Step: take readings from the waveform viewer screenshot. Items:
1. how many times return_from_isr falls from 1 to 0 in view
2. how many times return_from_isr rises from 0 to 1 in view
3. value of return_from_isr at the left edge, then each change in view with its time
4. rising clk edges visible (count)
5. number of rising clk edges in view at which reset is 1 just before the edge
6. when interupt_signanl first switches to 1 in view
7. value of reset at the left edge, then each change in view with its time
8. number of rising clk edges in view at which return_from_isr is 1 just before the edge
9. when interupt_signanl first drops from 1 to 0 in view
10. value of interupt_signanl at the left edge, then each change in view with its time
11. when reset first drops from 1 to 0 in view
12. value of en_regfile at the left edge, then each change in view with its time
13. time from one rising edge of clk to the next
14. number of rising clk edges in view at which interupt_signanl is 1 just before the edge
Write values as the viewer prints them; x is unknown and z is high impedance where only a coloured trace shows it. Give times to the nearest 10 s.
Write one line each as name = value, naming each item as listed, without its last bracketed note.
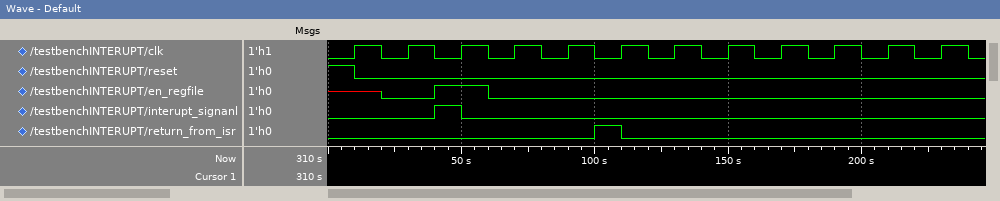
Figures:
how many times return_from_isr falls from 1 to 0 in view = 1
how many times return_from_isr rises from 0 to 1 in view = 1
value of return_from_isr at the left edge, then each change in view with its time = 0, 1 at 100 s, 0 at 110 s
rising clk edges visible = 12
number of rising clk edges in view at which reset is 1 just before the edge = 1
when interupt_signanl first switches to 1 in view = 40 s
value of reset at the left edge, then each change in view with its time = 1, 0 at 10 s
number of rising clk edges in view at which return_from_isr is 1 just before the edge = 1
when interupt_signanl first drops from 1 to 0 in view = 50 s
value of interupt_signanl at the left edge, then each change in view with its time = 0, 1 at 40 s, 0 at 50 s
when reset first drops from 1 to 0 in view = 10 s
value of en_regfile at the left edge, then each change in view with its time = x, 0 at 20 s, 1 at 40 s, 0 at 60 s
time from one rising edge of clk to the next = 20 s
number of rising clk edges in view at which interupt_signanl is 1 just before the edge = 1
